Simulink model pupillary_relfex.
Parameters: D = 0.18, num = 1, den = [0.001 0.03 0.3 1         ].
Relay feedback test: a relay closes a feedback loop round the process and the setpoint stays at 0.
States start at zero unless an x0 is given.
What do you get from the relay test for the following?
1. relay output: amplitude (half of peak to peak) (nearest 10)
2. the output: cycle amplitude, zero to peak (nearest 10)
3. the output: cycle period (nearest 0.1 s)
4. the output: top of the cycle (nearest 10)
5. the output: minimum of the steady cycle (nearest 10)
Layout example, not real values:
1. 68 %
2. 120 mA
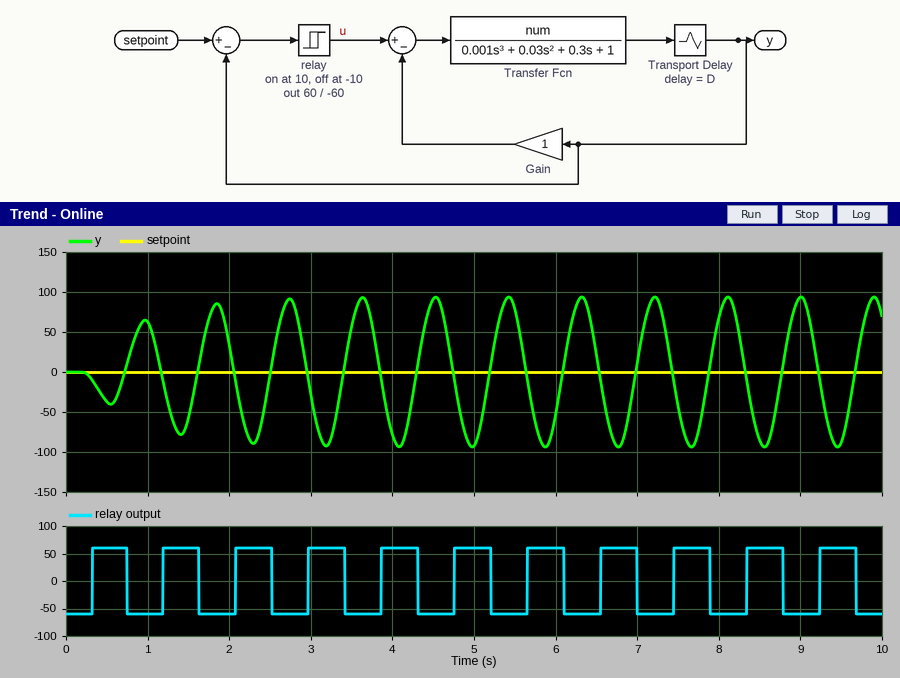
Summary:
1. 60
2. 90
3. 0.9 s
4. 90
5. -90
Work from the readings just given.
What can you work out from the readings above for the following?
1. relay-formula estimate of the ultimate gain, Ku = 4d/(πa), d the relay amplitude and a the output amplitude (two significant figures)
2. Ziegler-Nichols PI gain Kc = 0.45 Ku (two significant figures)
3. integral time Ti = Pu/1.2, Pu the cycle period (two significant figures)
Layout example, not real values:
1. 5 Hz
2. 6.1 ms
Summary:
1. 0.85
2. 0.38
3. 0.75 s
